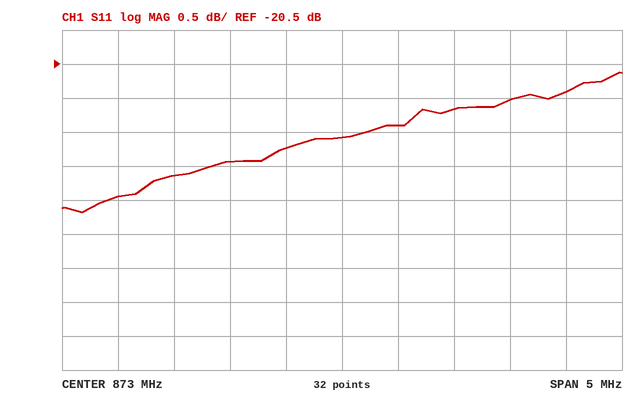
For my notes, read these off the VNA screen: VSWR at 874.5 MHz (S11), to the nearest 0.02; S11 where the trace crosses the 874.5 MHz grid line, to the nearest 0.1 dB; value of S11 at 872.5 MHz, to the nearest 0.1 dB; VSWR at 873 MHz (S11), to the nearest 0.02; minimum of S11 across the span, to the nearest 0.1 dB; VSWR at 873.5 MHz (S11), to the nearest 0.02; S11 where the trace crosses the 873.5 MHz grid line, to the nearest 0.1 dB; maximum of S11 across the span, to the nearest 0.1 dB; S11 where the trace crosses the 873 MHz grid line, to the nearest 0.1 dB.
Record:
1.20
-21.0 dB
-21.7 dB
1.18
-22.7 dB
1.18
-21.4 dB
-20.6 dB
-21.6 dB
